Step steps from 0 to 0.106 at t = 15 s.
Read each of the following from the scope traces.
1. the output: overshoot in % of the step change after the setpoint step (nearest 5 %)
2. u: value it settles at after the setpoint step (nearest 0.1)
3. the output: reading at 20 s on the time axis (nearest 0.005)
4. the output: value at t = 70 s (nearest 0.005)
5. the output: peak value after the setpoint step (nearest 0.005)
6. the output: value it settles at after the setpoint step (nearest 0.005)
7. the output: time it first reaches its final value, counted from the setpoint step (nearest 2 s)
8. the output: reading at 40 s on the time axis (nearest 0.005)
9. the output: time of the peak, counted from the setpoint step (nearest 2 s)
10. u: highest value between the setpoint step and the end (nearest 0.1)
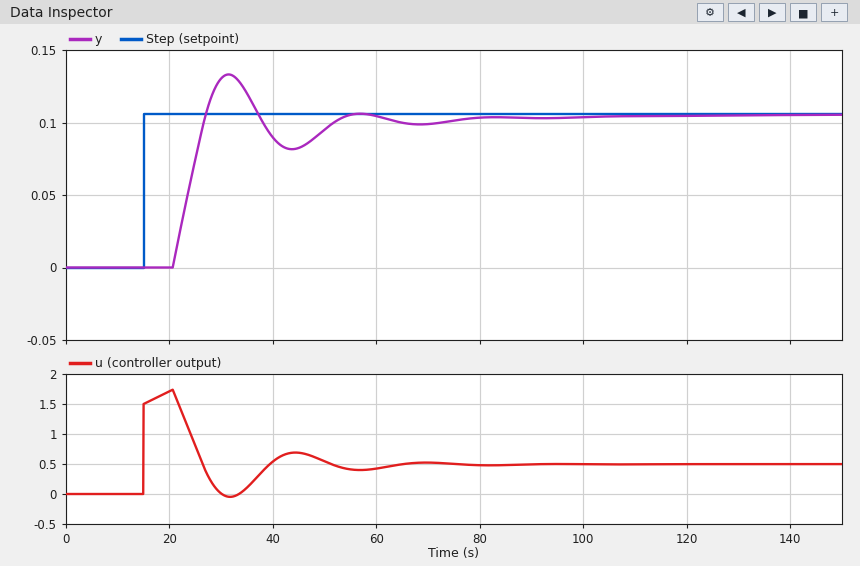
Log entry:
25 %
0.5
0.000
0.100
0.135
0.105
12 s
0.090
16 s
1.7
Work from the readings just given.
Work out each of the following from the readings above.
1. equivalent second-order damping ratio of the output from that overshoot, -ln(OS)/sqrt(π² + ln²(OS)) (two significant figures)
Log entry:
0.40
